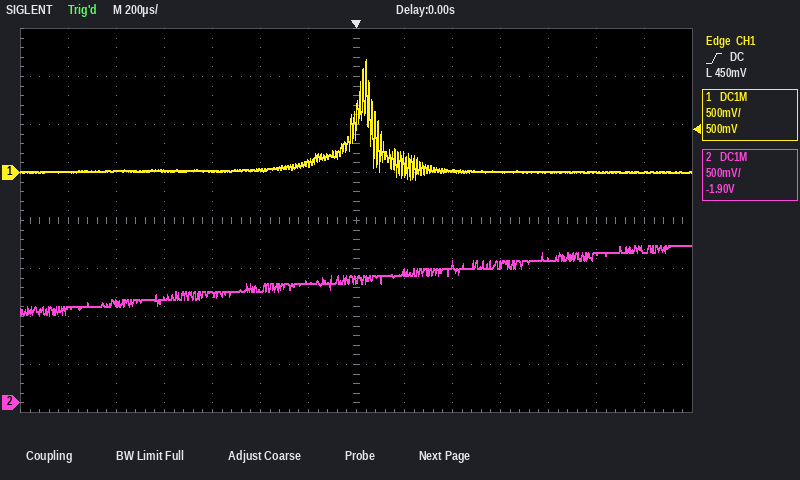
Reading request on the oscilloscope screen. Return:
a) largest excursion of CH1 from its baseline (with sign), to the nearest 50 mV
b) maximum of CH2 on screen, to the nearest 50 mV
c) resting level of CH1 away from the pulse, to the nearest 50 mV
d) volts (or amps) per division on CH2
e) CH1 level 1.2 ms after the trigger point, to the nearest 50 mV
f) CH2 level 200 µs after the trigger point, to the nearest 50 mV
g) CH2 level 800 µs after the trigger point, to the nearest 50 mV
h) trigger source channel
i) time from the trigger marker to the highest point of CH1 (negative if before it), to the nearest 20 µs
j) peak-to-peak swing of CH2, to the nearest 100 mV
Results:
+1.15 V
1.65 V
0 mV
500 mV
0 mV
1.35 V
1.50 V
CH1
+40 µs
700 mV
